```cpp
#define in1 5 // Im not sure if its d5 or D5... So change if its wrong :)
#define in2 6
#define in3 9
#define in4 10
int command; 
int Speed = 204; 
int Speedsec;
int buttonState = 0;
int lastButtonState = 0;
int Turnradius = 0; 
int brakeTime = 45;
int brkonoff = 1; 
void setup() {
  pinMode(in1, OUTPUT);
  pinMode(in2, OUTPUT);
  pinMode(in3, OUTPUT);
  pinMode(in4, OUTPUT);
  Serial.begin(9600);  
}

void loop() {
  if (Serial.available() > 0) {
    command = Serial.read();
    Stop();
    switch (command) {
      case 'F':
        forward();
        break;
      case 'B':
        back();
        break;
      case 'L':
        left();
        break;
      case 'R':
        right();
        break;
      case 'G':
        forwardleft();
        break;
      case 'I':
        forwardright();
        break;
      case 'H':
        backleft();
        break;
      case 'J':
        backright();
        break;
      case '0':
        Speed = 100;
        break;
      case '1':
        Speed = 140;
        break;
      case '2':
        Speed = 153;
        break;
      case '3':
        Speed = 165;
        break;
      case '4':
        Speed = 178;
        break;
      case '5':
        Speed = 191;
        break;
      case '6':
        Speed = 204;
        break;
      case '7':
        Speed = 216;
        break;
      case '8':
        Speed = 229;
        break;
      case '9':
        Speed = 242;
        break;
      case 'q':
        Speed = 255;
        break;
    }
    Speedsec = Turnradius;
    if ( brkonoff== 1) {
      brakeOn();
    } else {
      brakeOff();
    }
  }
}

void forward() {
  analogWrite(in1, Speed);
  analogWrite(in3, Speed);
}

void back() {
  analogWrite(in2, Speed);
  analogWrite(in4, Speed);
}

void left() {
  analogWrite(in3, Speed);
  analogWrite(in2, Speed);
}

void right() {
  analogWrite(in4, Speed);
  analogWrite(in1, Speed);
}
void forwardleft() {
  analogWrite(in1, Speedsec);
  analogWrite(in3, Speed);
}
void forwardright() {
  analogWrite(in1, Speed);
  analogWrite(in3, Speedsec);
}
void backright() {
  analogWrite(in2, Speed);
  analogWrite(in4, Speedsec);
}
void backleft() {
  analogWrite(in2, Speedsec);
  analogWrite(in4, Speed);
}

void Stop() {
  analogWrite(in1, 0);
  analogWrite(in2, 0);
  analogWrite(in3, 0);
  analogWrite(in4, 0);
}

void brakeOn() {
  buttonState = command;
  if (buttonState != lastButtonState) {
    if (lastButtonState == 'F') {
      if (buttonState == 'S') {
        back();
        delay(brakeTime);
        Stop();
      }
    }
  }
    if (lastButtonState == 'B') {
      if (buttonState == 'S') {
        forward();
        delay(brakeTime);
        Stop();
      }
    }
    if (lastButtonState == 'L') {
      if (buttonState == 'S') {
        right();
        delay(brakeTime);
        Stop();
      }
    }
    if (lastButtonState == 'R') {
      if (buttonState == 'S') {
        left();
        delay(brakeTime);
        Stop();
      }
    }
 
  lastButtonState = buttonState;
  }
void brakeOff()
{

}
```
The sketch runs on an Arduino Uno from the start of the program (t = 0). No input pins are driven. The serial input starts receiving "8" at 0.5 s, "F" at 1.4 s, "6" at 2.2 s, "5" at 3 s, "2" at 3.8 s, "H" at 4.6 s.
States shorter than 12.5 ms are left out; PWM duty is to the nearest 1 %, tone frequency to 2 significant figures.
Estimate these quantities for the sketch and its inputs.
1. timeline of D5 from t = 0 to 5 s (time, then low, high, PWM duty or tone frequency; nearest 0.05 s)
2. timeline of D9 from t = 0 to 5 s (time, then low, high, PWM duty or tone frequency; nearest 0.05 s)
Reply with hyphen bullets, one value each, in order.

- 0 s low; 1.4 s PWM 90 %; 2.2 s low
- 0 s low; 1.4 s PWM 90 %; 2.2 s low
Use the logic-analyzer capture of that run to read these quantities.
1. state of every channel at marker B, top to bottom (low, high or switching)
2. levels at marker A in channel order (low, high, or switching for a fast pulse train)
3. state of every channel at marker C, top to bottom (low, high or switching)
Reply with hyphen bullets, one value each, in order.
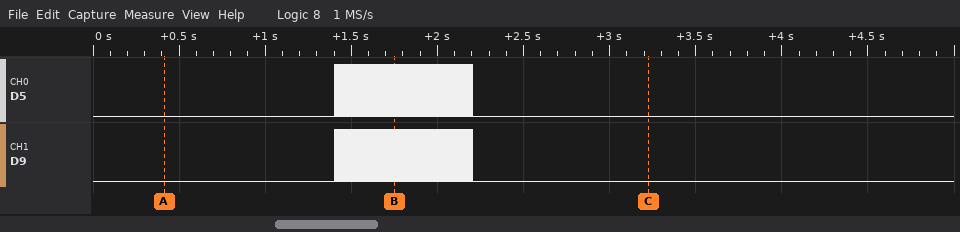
- D5 switching, D9 switching
- D5 low, D9 low
- D5 low, D9 low
